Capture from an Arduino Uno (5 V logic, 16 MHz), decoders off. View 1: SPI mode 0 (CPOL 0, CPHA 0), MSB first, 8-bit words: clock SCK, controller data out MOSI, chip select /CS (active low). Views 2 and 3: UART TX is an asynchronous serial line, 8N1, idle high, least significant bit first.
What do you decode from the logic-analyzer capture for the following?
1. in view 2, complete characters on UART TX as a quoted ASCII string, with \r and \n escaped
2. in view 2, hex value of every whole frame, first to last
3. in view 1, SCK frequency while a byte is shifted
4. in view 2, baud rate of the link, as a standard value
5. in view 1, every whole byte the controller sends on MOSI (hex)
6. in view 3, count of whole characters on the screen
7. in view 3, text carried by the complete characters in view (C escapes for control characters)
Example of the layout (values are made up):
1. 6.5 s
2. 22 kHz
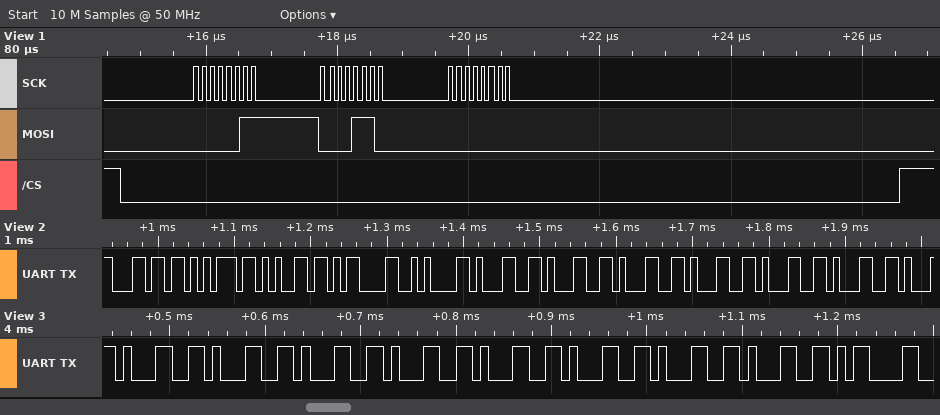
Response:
1. "lue\r\n111111"
2. 6C 75 65 0D 0A 31 31 31 31 31 31
3. 8 MHz
4. 115200 baud
5. 0x03 0x0E 0x00
6. 9
7. "11111111\r"
